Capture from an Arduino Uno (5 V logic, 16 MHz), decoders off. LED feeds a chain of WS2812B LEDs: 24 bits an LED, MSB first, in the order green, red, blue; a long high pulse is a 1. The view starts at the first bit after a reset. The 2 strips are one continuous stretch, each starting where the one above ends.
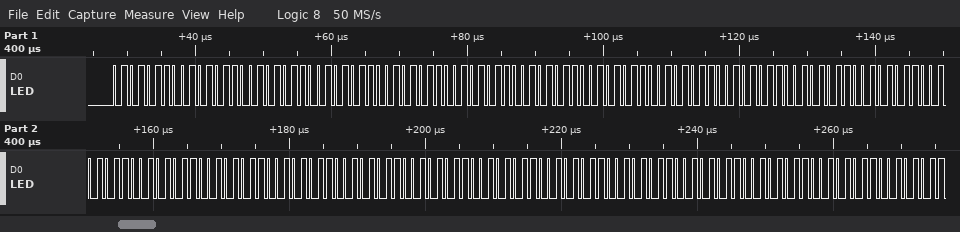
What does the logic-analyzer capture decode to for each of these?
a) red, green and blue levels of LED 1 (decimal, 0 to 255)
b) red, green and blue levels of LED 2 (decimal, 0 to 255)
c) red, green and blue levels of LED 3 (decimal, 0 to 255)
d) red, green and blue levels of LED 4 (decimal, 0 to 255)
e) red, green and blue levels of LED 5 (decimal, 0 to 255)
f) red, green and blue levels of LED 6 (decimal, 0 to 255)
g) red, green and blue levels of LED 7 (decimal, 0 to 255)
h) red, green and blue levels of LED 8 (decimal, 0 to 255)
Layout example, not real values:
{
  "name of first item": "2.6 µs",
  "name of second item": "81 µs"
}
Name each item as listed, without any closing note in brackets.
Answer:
{
  "red, green and blue levels of LED 1": "86, 86, 86",
  "red, green and blue levels of LED 2": "86, 86, 86",
  "red, green and blue levels of LED 3": "86, 86, 86",
  "red, green and blue levels of LED 4": "86, 86, 86",
  "red, green and blue levels of LED 5": "86, 86, 86",
  "red, green and blue levels of LED 6": "86, 86, 86",
  "red, green and blue levels of LED 7": "86, 86, 86",
  "red, green and blue levels of LED 8": "86, 86, 86"
}
